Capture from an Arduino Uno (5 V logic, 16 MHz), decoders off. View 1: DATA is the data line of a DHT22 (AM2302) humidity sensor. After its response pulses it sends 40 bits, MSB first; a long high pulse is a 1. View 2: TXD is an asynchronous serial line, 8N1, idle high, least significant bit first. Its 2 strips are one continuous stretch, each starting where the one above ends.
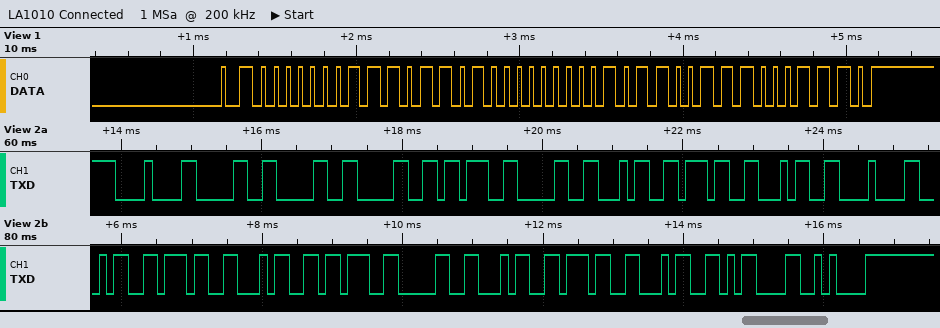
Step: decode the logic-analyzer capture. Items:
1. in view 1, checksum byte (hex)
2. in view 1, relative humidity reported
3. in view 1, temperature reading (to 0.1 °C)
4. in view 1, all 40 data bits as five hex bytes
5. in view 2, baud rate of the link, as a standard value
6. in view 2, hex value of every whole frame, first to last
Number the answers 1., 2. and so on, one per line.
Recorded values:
1. 0x8E
2. 47.4 %
3. 17.9 °C
4. 01 DA 00 B3 8E
5. 9600 baud
6. 0x08 0x30 0x30 0x30 0x3B 0x30 0x34 0x37 0x34 0x08 0x34 0x37 0x34 0x3B 0x30 0x34 0x37 0x34 0x0D 0x0A
